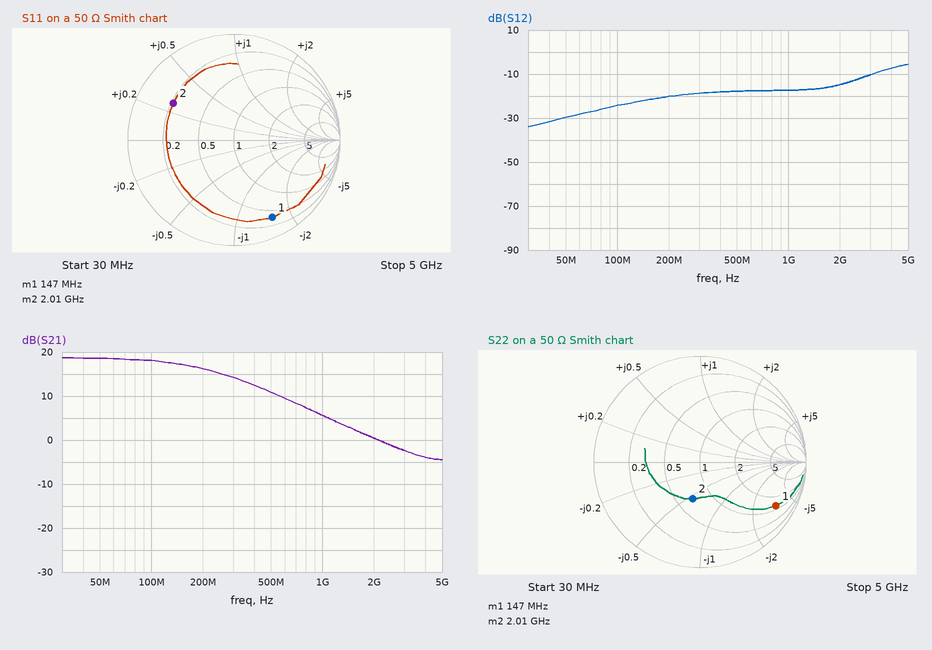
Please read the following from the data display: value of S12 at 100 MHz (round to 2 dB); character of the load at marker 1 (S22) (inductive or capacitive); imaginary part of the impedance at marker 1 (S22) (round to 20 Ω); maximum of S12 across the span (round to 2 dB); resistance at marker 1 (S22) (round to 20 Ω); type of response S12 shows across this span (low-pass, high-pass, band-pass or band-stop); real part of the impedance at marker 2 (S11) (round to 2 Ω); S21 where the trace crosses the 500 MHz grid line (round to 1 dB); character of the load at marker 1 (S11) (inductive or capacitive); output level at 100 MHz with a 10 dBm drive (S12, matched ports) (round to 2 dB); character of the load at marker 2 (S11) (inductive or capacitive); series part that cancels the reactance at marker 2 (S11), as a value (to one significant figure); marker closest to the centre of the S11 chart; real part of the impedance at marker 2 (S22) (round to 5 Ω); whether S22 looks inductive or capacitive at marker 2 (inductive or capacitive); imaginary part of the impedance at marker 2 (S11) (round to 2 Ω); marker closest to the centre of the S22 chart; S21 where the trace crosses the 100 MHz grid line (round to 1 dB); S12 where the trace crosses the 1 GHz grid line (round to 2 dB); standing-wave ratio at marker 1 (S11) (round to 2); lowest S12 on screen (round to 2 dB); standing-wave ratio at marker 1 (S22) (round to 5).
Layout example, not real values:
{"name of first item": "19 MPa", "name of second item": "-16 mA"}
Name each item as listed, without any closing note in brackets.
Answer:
{"value of S12 at 100 MHz": "-24 dB", "character of the load at marker 1 (S22)": "capacitive", "imaginary part of the impedance at marker 1 (S22)": "-160 Ω", "maximum of S12 across the span": "-6 dB", "resistance at marker 1 (S22)": "60 Ω", "type of response S12 shows across this span": "high-pass", "real part of the impedance at marker 2 (S11)": "10 Ω", "S21 where the trace crosses the 500 MHz grid line": "11 dB", "character of the load at marker 1 (S11)": "capacitive", "output level at 100 MHz with a 10 dBm drive (S12, matched ports)": "-14 dBm", "character of the load at marker 2 (S11)": "inductive", "series part that cancels the reactance at marker 2 (S11), as a value": "6 pF", "marker closest to the centre of the S11 chart": "marker 2", "real part of the impedance at marker 2 (S22)": "35 Ω", "whether S22 looks inductive or capacitive at marker 2": "capacitive", "imaginary part of the impedance at marker 2 (S11)": "+14 Ω", "marker closest to the centre of the S22 chart": "marker 2", "S21 where the trace crosses the 100 MHz grid line": "18 dB", "S12 where the trace crosses the 1 GHz grid line": "-18 dB", "standing-wave ratio at marker 1 (S11)": "10", "lowest S12 on screen": "-34 dB", "standing-wave ratio at marker 1 (S22)": "10"}
